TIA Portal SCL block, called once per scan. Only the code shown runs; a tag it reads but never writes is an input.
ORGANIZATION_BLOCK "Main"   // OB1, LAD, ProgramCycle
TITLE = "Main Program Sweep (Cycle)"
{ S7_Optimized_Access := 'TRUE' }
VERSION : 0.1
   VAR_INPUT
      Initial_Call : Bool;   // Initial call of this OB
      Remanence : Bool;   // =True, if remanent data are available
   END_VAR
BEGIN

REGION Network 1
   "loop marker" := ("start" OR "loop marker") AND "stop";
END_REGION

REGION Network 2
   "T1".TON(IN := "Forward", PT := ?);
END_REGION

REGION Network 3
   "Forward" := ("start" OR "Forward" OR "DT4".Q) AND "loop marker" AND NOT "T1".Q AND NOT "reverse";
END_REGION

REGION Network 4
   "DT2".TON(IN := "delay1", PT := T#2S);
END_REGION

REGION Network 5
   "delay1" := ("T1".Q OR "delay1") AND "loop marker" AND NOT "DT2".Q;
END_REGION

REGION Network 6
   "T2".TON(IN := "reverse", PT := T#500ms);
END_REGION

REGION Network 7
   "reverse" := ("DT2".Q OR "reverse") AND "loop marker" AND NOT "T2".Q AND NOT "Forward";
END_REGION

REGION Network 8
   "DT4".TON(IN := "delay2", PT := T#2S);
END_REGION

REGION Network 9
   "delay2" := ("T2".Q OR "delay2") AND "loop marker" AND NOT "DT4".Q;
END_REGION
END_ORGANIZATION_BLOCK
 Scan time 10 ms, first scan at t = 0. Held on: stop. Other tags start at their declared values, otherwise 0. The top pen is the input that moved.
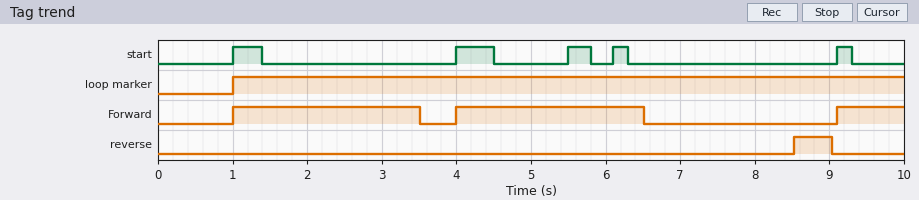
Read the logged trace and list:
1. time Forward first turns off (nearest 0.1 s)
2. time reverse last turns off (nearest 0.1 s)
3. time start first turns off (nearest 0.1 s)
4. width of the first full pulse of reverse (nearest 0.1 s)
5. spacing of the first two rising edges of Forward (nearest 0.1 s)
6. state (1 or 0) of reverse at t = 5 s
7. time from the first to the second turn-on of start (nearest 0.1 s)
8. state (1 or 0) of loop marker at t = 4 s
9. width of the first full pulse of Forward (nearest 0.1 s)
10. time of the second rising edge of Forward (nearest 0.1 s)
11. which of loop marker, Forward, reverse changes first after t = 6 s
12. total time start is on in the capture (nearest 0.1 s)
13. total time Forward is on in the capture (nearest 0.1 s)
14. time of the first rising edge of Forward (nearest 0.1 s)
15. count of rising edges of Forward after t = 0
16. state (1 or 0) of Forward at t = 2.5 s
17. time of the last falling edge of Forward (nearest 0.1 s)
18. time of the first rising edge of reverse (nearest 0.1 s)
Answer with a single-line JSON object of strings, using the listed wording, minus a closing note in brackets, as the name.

{"time Forward first turns off": "3.5 s", "time reverse last turns off": "9.0 s", "time start first turns off": "1.4 s", "width of the first full pulse of reverse": "0.5 s", "spacing of the first two rising edges of Forward": "3.0 s", "state (1 or 0) of reverse at t = 5 s": "0", "time from the first to the second turn-on of start": "3.0 s", "state (1 or 0) of loop marker at t = 4 s": "1", "width of the first full pulse of Forward": "2.5 s", "time of the second rising edge of Forward": "4.0 s", "which of loop marker, Forward, reverse changes first after t = 6 s": "Forward", "total time start is on in the capture": "1.6 s", "total time Forward is on in the capture": "5.9 s", "time of the first rising edge of Forward": "1.0 s", "count of rising edges of Forward after t = 0": "3", "state (1 or 0) of Forward at t = 2.5 s": "1", "time of the last falling edge of Forward": "6.5 s", "time of the first rising edge of reverse": "8.5 s"}
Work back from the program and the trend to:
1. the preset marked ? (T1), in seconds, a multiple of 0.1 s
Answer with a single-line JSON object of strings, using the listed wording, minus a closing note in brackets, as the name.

{"the preset marked ? (T1), in seconds, a multiple of 0.1 s": "2.5 s"}
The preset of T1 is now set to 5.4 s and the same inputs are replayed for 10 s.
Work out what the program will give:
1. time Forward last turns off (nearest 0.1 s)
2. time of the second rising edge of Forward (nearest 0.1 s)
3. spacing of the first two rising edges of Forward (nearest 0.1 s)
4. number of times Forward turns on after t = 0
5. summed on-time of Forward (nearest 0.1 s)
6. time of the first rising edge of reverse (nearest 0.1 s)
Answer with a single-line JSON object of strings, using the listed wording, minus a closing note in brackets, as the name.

{"time Forward last turns off": "6.4 s", "time of the second rising edge of Forward": "9.1 s", "spacing of the first two rising edges of Forward": "8.1 s", "number of times Forward turns on after t = 0": "2", "summed on-time of Forward": "6.3 s", "time of the first rising edge of reverse": "8.4 s"}
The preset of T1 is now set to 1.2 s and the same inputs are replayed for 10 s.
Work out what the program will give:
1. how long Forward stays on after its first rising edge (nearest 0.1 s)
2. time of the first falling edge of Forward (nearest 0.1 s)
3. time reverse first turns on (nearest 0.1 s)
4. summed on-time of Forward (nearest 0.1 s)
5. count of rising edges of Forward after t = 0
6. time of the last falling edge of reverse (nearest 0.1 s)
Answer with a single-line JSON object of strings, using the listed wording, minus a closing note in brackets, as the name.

{"how long Forward stays on after its first rising edge": "1.2 s", "time of the first falling edge of Forward": "2.2 s", "time reverse first turns on": "7.2 s", "summed on-time of Forward": "4.5 s", "count of rising edges of Forward after t = 0": "4", "time of the last falling edge of reverse": "7.7 s"}
